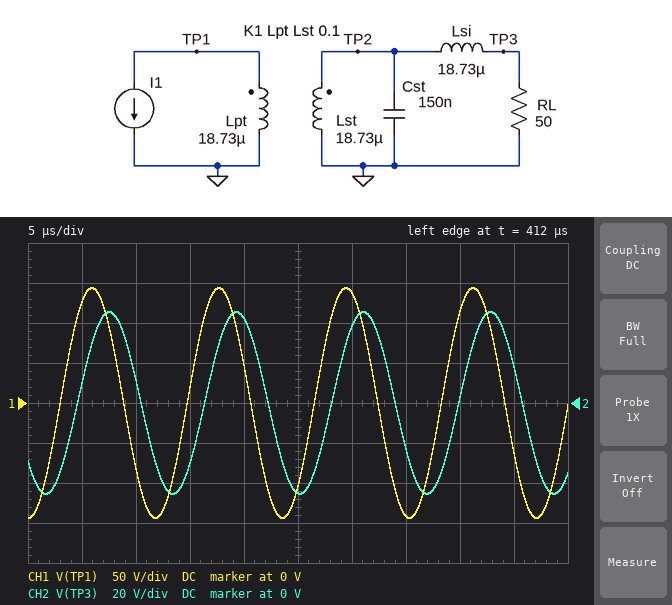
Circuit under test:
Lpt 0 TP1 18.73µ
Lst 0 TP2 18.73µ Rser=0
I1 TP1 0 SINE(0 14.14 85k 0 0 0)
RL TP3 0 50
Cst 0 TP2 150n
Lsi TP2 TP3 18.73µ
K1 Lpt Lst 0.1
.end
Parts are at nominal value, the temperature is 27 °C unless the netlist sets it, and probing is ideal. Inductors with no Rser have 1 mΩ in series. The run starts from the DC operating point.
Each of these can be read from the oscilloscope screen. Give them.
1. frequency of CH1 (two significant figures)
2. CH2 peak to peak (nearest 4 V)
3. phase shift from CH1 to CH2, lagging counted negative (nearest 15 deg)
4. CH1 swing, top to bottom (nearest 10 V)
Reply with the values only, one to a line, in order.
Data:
85 kHz
92 V
-45 deg
290 V
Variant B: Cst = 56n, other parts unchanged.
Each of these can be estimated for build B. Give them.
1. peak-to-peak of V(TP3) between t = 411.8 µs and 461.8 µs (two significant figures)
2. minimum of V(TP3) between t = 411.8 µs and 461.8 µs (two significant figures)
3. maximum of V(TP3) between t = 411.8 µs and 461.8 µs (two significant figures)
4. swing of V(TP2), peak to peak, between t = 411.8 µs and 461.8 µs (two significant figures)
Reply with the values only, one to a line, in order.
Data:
36 V
-18 V
18 V
37 V
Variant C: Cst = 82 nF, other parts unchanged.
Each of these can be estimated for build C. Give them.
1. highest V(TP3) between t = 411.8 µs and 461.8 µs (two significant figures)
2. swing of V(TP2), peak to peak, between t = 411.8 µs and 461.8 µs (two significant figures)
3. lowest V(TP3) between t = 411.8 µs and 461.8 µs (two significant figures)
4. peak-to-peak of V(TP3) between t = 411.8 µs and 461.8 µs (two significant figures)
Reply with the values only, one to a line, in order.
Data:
22 V
45 V
-22 V
44 V
